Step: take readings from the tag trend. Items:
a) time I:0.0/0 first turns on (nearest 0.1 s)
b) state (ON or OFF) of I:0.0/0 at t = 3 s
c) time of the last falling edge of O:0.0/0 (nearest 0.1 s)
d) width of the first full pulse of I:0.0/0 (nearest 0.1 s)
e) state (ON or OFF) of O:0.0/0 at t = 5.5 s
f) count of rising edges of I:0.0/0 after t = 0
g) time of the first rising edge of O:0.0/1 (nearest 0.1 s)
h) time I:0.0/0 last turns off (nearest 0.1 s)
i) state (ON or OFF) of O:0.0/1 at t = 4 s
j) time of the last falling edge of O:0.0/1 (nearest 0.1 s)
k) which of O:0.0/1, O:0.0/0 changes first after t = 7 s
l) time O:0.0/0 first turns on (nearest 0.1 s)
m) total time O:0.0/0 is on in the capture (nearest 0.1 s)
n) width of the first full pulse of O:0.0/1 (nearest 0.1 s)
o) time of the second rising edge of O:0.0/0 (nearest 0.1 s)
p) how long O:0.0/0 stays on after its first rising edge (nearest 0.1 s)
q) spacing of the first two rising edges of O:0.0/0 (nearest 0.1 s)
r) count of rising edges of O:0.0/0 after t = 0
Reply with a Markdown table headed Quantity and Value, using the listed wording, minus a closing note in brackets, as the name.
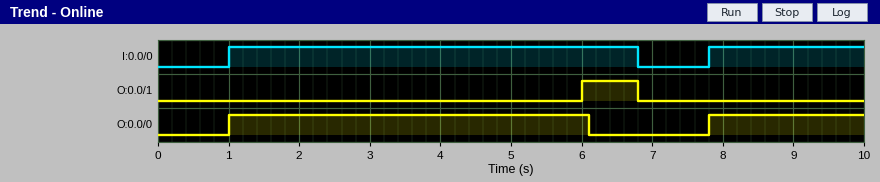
| Quantity | Value |
|---|---|
| time I:0.0/0 first turns on | 1.0 s |
| state (ON or OFF) of I:0.0/0 at t = 3 s | ON |
| time of the last falling edge of O:0.0/0 | 6.1 s |
| width of the first full pulse of I:0.0/0 | 5.8 s |
| state (ON or OFF) of O:0.0/0 at t = 5.5 s | ON |
| count of rising edges of I:0.0/0 after t = 0 | 2 |
| time of the first rising edge of O:0.0/1 | 6.0 s |
| time I:0.0/0 last turns off | 6.8 s |
| state (ON or OFF) of O:0.0/1 at t = 4 s | OFF |
| time of the last falling edge of O:0.0/1 | 6.8 s |
| which of O:0.0/1, O:0.0/0 changes first after t = 7 s | O:0.0/0 |
| time O:0.0/0 first turns on | 1.0 s |
| total time O:0.0/0 is on in the capture | 7.3 s |
| width of the first full pulse of O:0.0/1 | 0.8 s |
| time of the second rising edge of O:0.0/0 | 7.8 s |
| how long O:0.0/0 stays on after its first rising edge | 5.1 s |
| spacing of the first two rising edges of O:0.0/0 | 6.8 s |
| count of rising edges of O:0.0/0 after t = 0 | 2 |
